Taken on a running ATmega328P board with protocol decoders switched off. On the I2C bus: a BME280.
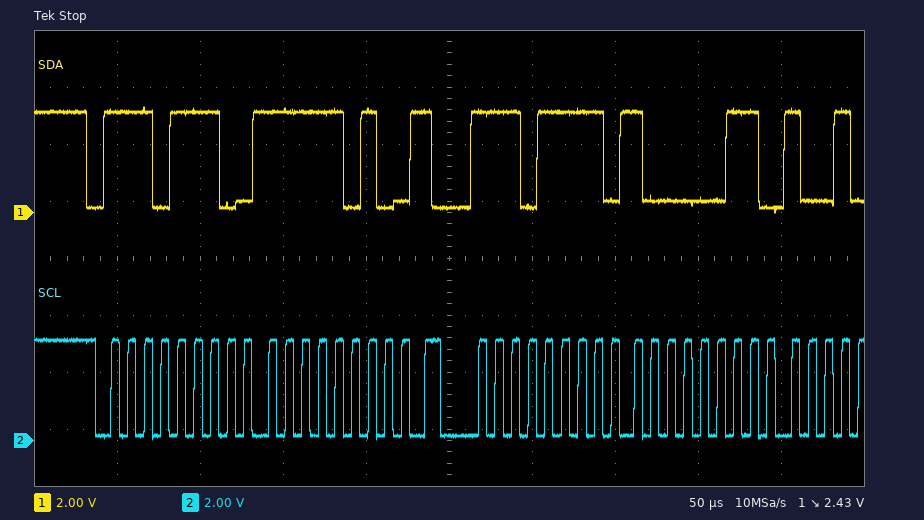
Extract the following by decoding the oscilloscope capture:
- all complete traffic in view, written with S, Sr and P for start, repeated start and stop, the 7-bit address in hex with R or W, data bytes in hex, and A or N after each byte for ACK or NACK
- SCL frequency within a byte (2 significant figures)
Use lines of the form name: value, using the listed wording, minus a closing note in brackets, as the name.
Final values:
all complete traffic in view, written with S, Sr and P for start, repeated start and stop, the 7-bit address in hex with R or W, data bytes in hex, and A or N after each byte for ACK or NACK: S 77W A FA A Sr 77R A 83 A
SCL frequency within a byte: 100 kHz
